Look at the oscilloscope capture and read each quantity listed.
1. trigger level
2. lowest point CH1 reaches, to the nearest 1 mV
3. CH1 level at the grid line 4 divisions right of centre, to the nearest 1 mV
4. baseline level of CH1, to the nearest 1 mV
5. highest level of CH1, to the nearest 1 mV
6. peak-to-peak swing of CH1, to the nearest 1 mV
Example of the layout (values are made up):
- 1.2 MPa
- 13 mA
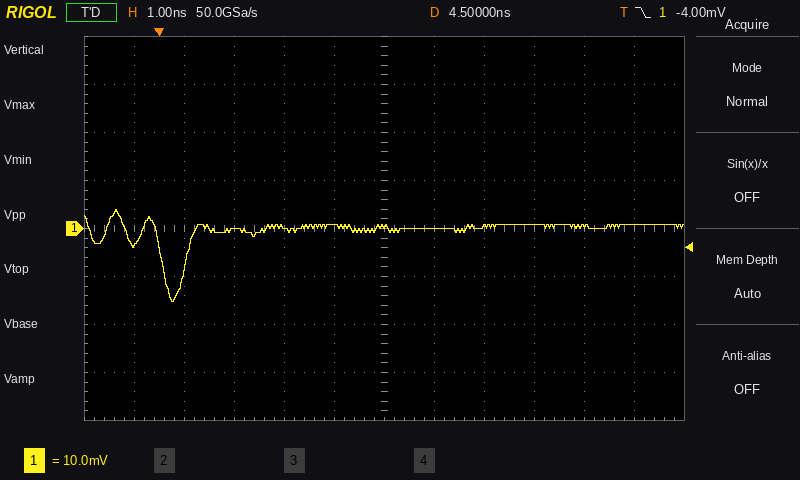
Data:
- -4.00 mV
- -15 mV
- 0 mV
- 0 mV
- 4 mV
- 19 mV
